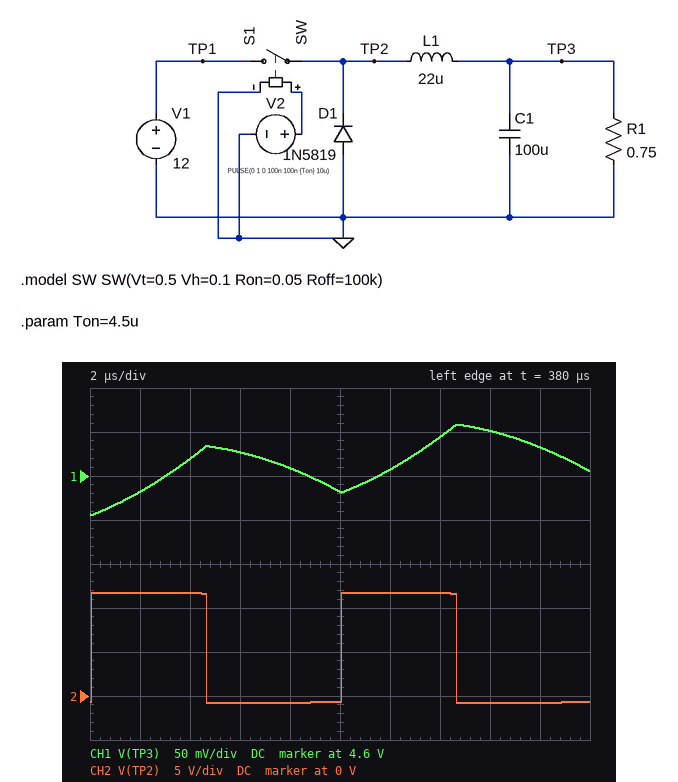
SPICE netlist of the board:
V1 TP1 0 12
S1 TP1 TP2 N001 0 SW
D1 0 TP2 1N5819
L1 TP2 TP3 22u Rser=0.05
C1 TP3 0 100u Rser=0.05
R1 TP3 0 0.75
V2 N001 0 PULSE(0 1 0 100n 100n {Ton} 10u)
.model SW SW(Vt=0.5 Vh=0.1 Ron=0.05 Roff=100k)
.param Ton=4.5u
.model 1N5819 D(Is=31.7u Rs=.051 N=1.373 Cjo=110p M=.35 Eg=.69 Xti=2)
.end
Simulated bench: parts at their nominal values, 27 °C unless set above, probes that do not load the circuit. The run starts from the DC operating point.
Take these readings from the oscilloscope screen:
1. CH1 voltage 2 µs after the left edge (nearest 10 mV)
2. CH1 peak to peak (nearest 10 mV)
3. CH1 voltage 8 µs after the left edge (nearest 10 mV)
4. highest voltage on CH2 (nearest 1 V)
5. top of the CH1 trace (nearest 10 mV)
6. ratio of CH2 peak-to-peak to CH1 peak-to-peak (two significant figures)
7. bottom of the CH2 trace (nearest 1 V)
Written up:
4.58 V
100 mV
4.61 V
12 V
4.66 V
120
-1 V
